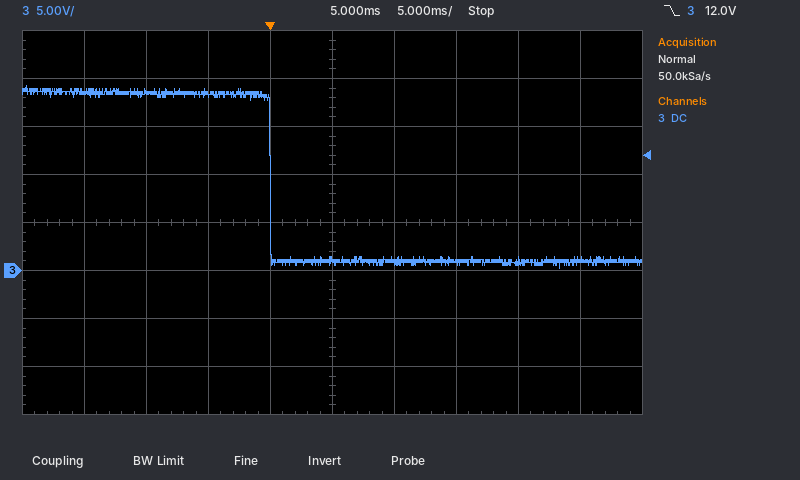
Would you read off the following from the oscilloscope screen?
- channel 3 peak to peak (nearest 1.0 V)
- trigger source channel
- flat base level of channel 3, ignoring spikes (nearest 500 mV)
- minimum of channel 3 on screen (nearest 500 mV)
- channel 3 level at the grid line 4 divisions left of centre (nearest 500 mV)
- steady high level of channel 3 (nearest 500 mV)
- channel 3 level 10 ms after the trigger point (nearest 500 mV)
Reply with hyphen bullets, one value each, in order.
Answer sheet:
- 19.0 V
- channel 3
- 1.0 V
- 0.0 V
- 18.5 V
- 18.5 V
- 1.0 V
